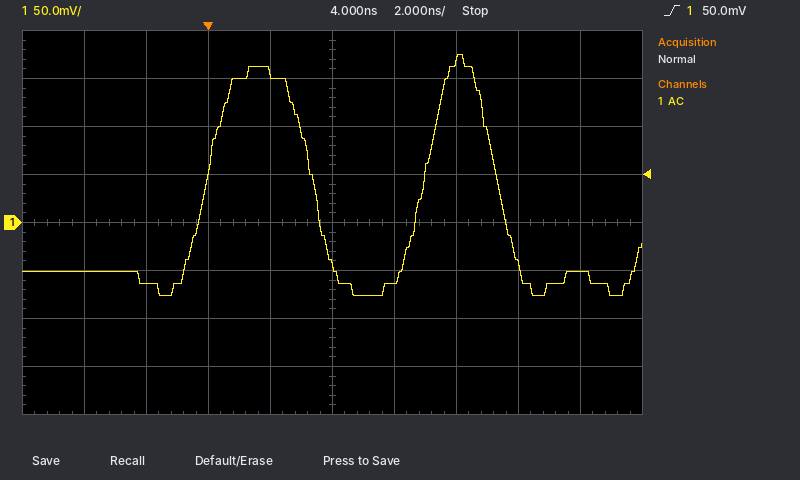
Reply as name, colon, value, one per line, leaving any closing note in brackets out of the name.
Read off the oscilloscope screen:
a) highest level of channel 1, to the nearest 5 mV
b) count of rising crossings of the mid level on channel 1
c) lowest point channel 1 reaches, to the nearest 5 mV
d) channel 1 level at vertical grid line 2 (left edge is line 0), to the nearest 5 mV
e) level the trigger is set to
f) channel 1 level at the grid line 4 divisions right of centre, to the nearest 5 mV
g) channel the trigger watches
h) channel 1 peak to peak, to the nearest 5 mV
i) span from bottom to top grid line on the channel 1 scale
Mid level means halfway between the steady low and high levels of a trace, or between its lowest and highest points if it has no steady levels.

highest level of channel 1, to the nearest 5 mV: 175 mV
count of rising crossings of the mid level on channel 1: 2
lowest point channel 1 reaches, to the nearest 5 mV: -75 mV
channel 1 level at vertical grid line 2 (left edge is line 0), to the nearest 5 mV: -65 mV
level the trigger is set to: 50.0 mV
channel 1 level at the grid line 4 divisions right of centre, to the nearest 5 mV: -50 mV
channel the trigger watches: channel 1
channel 1 peak to peak, to the nearest 5 mV: 250 mV
span from bottom to top grid line on the channel 1 scale: 400 mV
